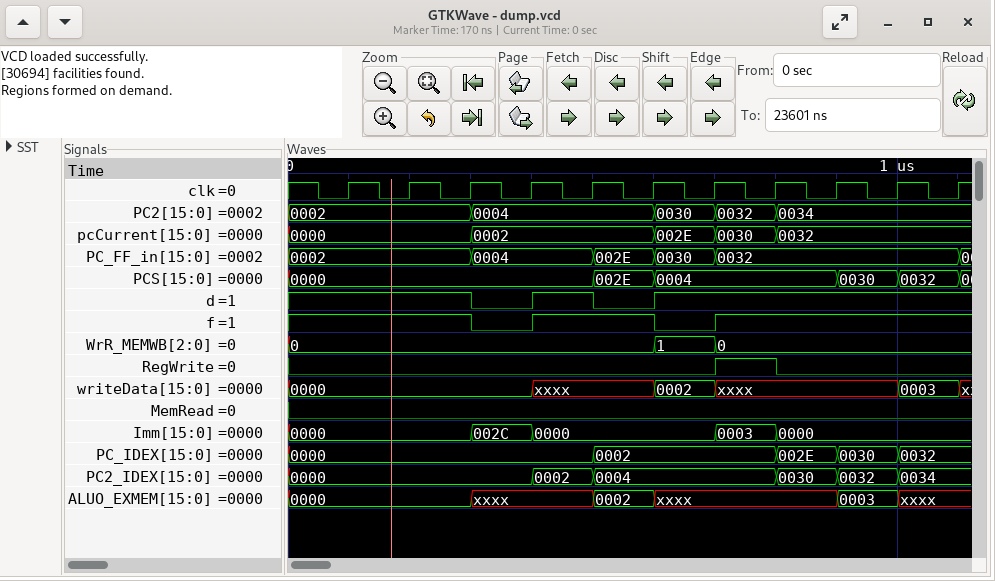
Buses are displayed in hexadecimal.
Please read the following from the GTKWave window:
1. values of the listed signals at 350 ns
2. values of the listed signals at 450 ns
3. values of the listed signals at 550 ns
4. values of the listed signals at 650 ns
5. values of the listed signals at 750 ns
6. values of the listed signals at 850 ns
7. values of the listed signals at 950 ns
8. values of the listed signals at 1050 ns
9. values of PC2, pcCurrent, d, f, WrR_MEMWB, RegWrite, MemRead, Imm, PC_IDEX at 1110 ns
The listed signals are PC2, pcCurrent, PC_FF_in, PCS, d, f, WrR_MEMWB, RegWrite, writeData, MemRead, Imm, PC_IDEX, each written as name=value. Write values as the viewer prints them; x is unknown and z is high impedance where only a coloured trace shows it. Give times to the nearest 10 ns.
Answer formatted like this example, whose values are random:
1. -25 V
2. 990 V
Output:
1. PC2=0004, pcCurrent=0002, PC_FF_in=0004, PCS=0000, d=0, f=0, WrR_MEMWB=0, RegWrite=0, writeData=0000, MemRead=0, Imm=002C, PC_IDEX=0000
2. PC2=0004, pcCurrent=0002, PC_FF_in=0004, PCS=0000, d=1, f=1, WrR_MEMWB=0, RegWrite=0, writeData=xxxx, MemRead=0, Imm=0000, PC_IDEX=0000
3. PC2=0004, pcCurrent=0002, PC_FF_in=002E, PCS=002E, d=0, f=1, WrR_MEMWB=0, RegWrite=0, writeData=xxxx, MemRead=0, Imm=0000, PC_IDEX=0002
4. PC2=0030, pcCurrent=002E, PC_FF_in=0030, PCS=0004, d=1, f=0, WrR_MEMWB=1, RegWrite=0, writeData=0002, MemRead=0, Imm=0000, PC_IDEX=0002
5. PC2=0032, pcCurrent=0030, PC_FF_in=0032, PCS=0004, d=1, f=1, WrR_MEMWB=0, RegWrite=1, writeData=xxxx, MemRead=0, Imm=0003, PC_IDEX=0002
6. PC2=0034, pcCurrent=0032, PC_FF_in=0032, PCS=0004, d=1, f=1, WrR_MEMWB=0, RegWrite=0, writeData=xxxx, MemRead=0, Imm=0000, PC_IDEX=002E
7. PC2=0034, pcCurrent=0032, PC_FF_in=0032, PCS=0030, d=1, f=1, WrR_MEMWB=0, RegWrite=0, writeData=xxxx, MemRead=0, Imm=0000, PC_IDEX=0030
8. PC2=0034, pcCurrent=0032, PC_FF_in=0032, PCS=0032, d=1, f=1, WrR_MEMWB=0, RegWrite=0, writeData=0003, MemRead=0, Imm=0000, PC_IDEX=0032
9. PC2=0034, pcCurrent=0032, d=1, f=1, WrR_MEMWB=0, RegWrite=0, MemRead=0, Imm=0000, PC_IDEX=0032
